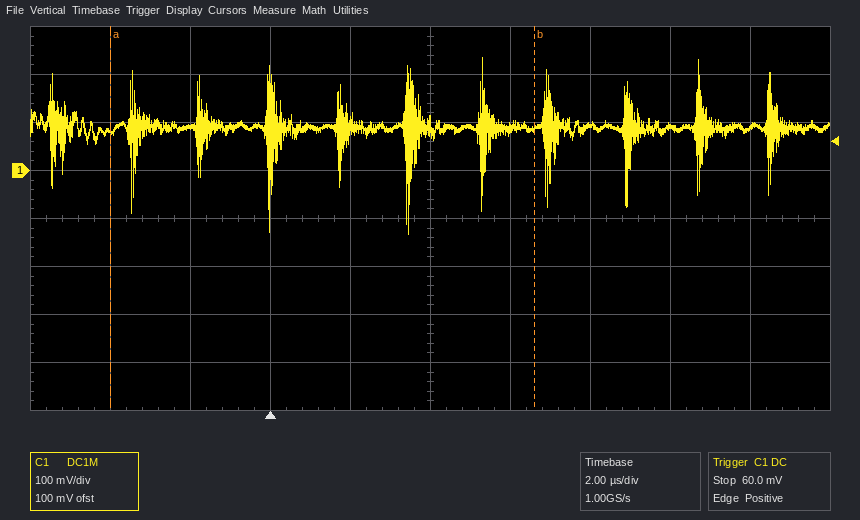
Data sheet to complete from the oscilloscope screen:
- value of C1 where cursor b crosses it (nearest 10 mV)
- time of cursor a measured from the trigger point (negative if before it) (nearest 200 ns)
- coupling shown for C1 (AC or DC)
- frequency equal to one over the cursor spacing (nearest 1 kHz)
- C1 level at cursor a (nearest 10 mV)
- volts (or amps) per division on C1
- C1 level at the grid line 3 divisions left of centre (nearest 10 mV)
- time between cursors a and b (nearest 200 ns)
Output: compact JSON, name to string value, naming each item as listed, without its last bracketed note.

{"value of C1 where cursor b crosses it": "90 mV", "time of cursor a measured from the trigger point (negative if before it)": "-4.0 µs", "coupling shown for C1": "DC", "frequency equal to one over the cursor spacing": "94 kHz", "C1 level at cursor a": "80 mV", "volts (or amps) per division on C1": "100 mV", "C1 level at the grid line 3 divisions left of centre": "90 mV", "time between cursors a and b": "10.6 µs"}
